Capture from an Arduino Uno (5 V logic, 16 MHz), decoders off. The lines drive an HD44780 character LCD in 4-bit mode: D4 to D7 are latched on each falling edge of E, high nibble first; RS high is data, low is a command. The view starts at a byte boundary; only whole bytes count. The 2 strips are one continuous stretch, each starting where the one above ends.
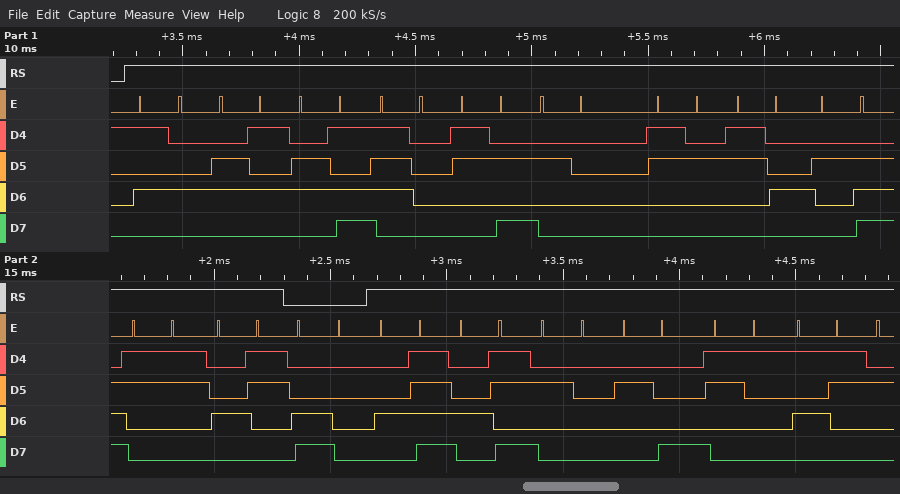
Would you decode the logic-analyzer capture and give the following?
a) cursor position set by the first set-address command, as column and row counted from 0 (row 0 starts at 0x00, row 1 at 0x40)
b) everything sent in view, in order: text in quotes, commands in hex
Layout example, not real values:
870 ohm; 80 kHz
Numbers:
column 0, row 1; "Temp: 24.3C" 0xC0 "OK (1S"
